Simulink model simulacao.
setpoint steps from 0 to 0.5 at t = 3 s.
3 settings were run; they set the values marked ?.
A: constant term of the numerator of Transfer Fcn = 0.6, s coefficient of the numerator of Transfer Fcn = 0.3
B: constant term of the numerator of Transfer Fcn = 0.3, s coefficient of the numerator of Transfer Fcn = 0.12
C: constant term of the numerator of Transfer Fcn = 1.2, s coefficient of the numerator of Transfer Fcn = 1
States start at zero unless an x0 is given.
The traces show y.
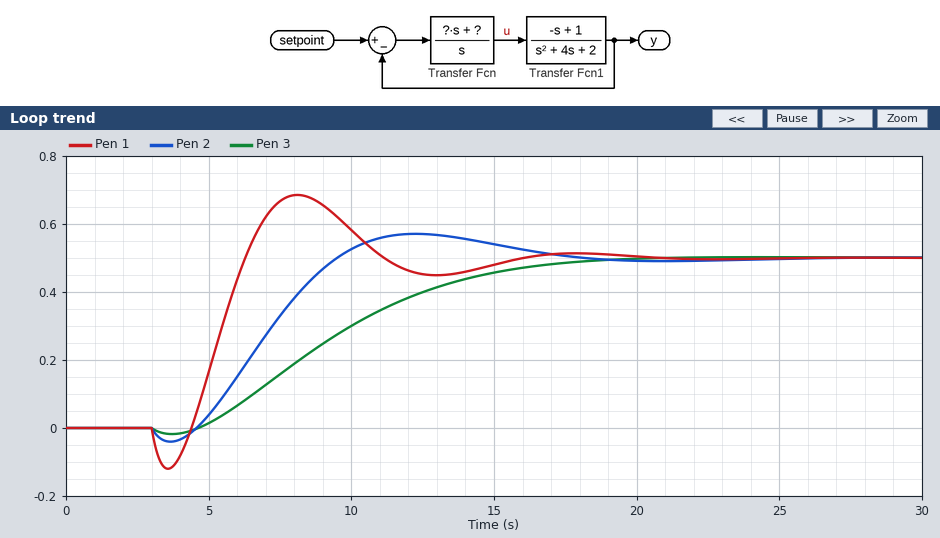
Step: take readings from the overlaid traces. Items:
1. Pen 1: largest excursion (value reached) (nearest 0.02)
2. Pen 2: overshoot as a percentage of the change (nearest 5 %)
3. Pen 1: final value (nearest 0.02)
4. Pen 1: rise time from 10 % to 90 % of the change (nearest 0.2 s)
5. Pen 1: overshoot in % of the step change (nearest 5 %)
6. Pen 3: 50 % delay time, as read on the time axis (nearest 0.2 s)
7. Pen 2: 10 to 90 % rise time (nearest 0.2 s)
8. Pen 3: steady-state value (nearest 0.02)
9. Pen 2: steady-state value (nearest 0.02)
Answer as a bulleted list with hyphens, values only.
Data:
- 0.68
- 15 %
- 0.50
- 1.4 s
- 35 %
- 9.0 s
- 3.6 s
- 0.50
- 0.50
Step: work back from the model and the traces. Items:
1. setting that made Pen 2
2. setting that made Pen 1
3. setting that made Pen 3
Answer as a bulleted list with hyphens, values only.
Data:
- A
- C
- B
